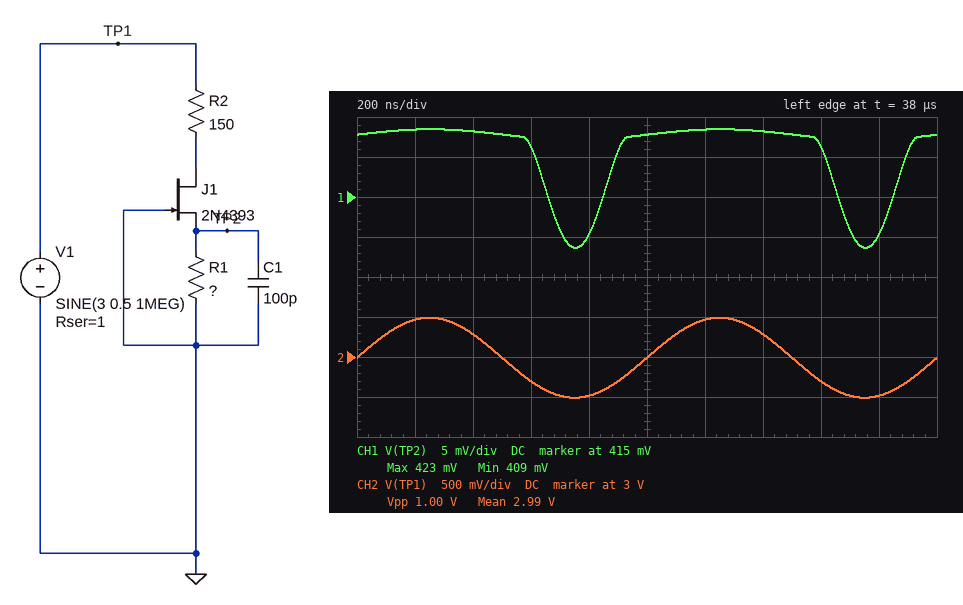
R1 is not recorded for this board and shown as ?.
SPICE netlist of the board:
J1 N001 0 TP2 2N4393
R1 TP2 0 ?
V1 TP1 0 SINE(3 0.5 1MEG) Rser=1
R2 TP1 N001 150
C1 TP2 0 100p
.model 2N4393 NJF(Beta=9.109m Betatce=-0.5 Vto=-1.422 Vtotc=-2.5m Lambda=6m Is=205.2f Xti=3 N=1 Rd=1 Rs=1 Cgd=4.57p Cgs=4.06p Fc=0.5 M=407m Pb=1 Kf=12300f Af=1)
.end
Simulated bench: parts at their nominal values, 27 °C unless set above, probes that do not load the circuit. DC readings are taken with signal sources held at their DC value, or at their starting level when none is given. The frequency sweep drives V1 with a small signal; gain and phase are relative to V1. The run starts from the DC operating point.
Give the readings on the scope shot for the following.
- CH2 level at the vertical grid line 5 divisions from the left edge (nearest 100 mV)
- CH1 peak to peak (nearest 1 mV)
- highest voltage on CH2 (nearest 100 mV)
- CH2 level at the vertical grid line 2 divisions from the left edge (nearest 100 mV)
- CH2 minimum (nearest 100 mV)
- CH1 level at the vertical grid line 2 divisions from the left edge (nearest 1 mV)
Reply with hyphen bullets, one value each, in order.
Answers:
- 3.0 V
- 15 mV
- 3.5 V
- 3.3 V
- 2.5 V
- 423 mV
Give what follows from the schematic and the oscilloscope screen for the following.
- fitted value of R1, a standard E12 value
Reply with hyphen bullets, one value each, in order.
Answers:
- 47 Ω
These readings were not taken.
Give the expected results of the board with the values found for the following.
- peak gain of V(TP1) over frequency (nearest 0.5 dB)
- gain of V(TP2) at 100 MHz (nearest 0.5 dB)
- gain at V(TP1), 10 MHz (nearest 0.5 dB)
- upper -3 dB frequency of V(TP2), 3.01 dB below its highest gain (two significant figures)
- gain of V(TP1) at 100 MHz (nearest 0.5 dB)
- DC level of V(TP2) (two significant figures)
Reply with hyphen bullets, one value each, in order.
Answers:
- 0 dB
- -63.5 dB
- 0 dB
- 59 MHz
- 0 dB
- 420 mV
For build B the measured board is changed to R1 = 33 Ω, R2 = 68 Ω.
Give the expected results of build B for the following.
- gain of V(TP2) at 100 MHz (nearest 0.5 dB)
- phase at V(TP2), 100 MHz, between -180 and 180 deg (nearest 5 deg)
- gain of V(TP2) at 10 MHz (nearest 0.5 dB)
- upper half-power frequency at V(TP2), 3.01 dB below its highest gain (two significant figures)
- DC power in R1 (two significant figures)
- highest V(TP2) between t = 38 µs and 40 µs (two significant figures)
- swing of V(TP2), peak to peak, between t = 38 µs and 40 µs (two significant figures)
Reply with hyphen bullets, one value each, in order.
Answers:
- -62.5 dB
- -60 deg
- -58.5 dB
- 76 MHz
- 3.6 mW
- 350 mV
- 1.2 mV
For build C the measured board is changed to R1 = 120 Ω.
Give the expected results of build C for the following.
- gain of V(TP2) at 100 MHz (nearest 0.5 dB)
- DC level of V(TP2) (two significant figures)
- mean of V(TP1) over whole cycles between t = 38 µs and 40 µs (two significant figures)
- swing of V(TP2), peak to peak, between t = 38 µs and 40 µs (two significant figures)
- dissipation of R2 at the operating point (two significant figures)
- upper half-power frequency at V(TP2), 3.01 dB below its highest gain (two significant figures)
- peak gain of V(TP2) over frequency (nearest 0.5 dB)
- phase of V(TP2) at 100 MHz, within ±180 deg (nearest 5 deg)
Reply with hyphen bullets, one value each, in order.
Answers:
- -67.0 dB
- 650 mV
- 3.0 V
- 1.4 mV
- 4.4 mW
- 34 MHz
- -57.0 dB
- -85 deg
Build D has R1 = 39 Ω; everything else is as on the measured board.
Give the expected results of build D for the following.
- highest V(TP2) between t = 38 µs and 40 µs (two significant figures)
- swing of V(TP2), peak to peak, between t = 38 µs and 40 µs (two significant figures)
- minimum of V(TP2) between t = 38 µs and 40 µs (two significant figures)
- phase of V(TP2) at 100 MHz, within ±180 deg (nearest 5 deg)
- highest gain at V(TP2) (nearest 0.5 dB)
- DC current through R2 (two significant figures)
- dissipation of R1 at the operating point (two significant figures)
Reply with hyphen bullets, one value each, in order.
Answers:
- 380 mV
- 22 mV
- 360 mV
- -70 deg
- -58.0 dB
- 9.8 mA
- 3.7 mW
